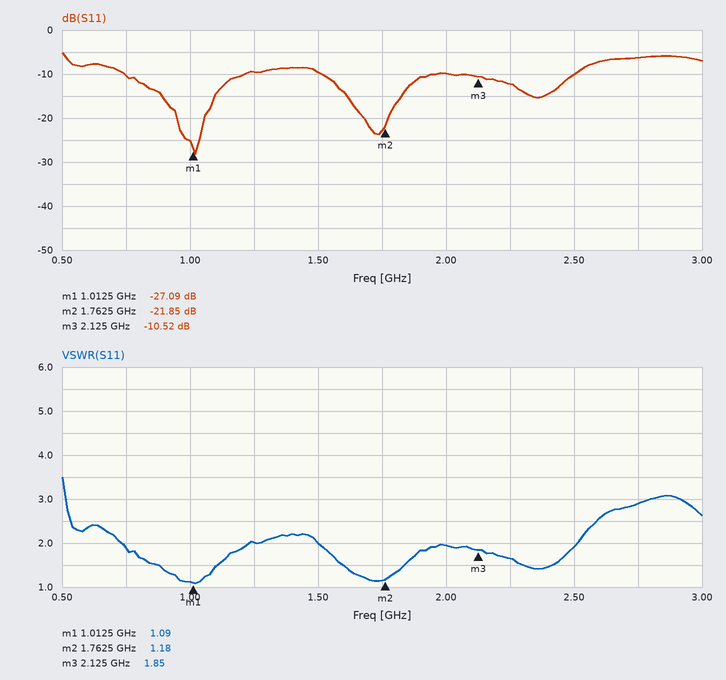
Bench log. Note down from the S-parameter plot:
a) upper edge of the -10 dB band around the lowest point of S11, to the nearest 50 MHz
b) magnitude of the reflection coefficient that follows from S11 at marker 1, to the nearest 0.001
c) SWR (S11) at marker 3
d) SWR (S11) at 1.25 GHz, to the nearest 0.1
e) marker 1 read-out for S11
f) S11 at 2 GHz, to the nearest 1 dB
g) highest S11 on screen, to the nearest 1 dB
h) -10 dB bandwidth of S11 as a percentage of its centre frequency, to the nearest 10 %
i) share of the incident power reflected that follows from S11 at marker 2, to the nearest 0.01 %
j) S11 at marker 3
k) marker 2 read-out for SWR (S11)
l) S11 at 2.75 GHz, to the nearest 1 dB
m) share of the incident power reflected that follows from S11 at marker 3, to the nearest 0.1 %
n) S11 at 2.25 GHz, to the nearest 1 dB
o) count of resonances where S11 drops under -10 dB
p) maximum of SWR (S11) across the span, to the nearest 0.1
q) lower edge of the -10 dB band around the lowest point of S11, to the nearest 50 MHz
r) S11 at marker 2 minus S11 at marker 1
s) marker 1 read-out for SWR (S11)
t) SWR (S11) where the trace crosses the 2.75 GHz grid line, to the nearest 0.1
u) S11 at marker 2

1.20 GHz
0.044
1.85
2.0
-27.09 dB
-10 dB
-5 dB
50 %
0.65 %
-10.52 dB
1.18
-6 dB
8.9 %
-12 dB
3
3.5
750 MHz
5.24 dB
1.09
2.9
-21.85 dB
